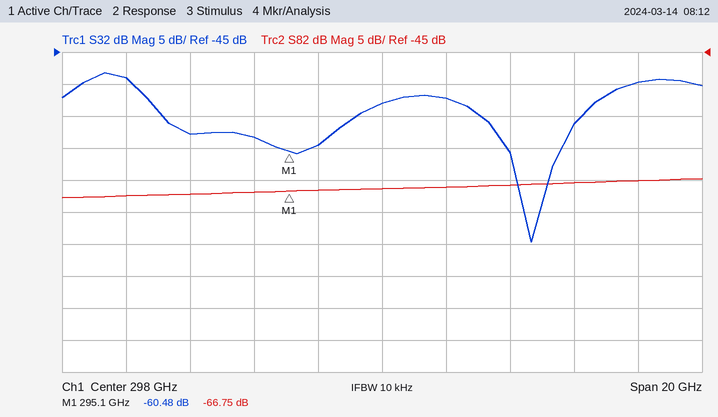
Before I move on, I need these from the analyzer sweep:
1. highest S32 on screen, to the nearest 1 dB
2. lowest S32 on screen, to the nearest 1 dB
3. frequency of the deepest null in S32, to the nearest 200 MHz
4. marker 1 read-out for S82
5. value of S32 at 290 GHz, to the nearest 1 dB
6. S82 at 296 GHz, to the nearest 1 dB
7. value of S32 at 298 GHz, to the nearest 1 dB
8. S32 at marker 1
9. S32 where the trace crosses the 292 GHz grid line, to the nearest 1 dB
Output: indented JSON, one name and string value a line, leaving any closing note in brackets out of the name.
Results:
{
  "highest S32 on screen, to the nearest 1 dB": "-48 dB",
  "lowest S32 on screen, to the nearest 1 dB": "-75 dB",
  "frequency of the deepest null in S32, to the nearest 200 MHz": "302.6 GHz",
  "marker 1 read-out for S82": "-66.75 dB",
  "value of S32 at 290 GHz, to the nearest 1 dB": "-49 dB",
  "S82 at 296 GHz, to the nearest 1 dB": "-67 dB",
  "value of S32 at 298 GHz, to the nearest 1 dB": "-53 dB",
  "S32 at marker 1": "-60.48 dB",
  "S32 where the trace crosses the 292 GHz grid line, to the nearest 1 dB": "-58 dB"
}
